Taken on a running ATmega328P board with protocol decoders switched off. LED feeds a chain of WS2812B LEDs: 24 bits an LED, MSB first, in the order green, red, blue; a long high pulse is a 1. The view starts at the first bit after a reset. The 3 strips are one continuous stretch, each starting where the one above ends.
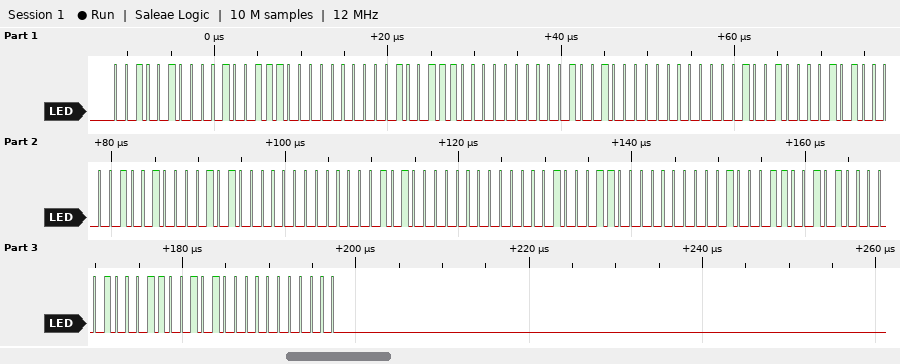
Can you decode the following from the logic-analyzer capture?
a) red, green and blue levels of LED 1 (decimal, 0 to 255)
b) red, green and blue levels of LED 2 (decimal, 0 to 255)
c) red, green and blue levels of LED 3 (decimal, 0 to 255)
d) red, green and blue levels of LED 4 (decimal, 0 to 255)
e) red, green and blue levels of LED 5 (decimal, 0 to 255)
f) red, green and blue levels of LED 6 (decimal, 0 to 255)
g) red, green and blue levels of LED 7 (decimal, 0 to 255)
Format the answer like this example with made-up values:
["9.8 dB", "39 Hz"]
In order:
["39, 36, 0", "0, 39, 36", "36, 0, 40", "40, 36, 0", "0, 40, 35", "35, 0, 40", "40, 35, 0"]
